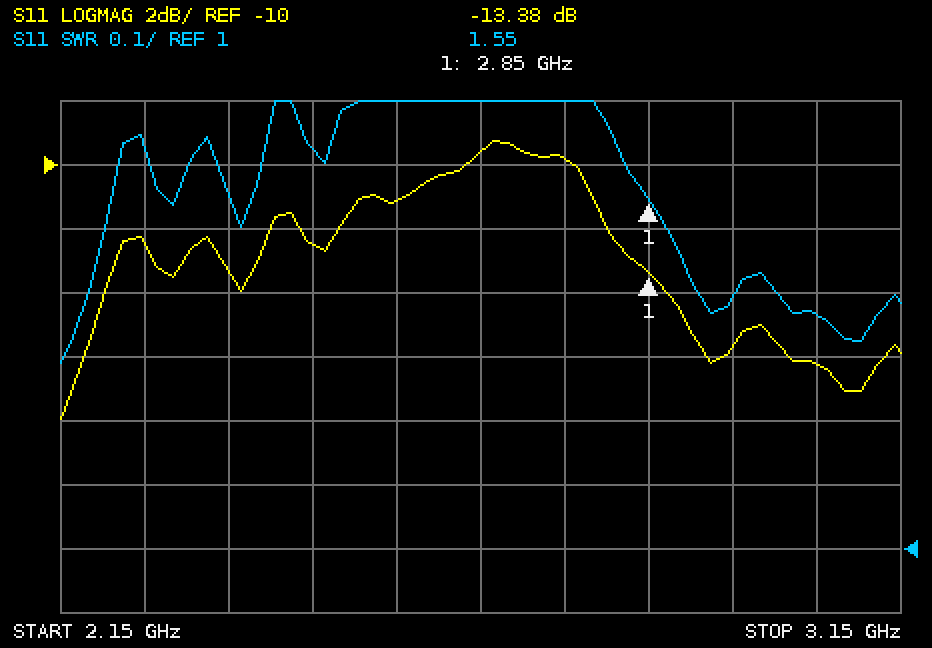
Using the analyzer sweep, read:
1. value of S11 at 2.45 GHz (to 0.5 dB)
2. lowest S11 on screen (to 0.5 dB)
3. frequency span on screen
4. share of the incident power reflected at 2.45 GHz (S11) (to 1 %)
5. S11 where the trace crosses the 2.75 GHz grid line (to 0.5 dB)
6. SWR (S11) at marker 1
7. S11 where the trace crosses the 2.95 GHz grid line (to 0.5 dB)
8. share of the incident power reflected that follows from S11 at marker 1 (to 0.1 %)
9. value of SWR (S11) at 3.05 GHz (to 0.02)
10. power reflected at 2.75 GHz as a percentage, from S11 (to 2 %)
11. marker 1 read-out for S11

-12.5 dB
-18.0 dB
1 GHz
6 %
-10.0 dB
1.55
-15.5 dB
4.6 %
1.36
10 %
-13.38 dB
